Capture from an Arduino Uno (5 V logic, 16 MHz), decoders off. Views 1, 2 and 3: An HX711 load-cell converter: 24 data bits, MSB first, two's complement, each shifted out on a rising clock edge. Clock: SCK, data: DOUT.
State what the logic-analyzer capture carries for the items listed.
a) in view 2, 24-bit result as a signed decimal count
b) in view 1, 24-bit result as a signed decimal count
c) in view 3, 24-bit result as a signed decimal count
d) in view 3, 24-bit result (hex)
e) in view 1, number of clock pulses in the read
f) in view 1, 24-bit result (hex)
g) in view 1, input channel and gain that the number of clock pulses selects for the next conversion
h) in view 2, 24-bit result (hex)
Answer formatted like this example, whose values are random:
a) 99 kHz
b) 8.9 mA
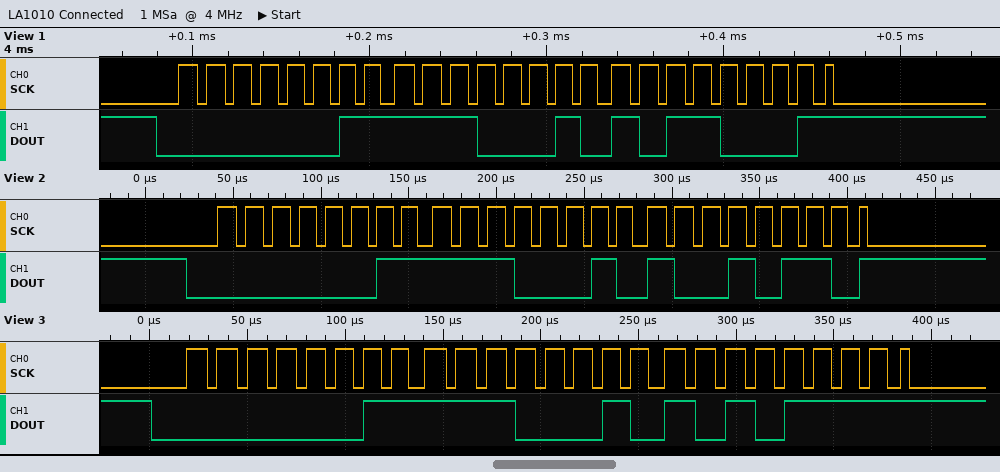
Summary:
a) 254614
b) 254641
c) 254639
d) 0x03E2AF
e) 25
f) 0x03E2B1
g) channel A, gain 128
h) 0x03E296
